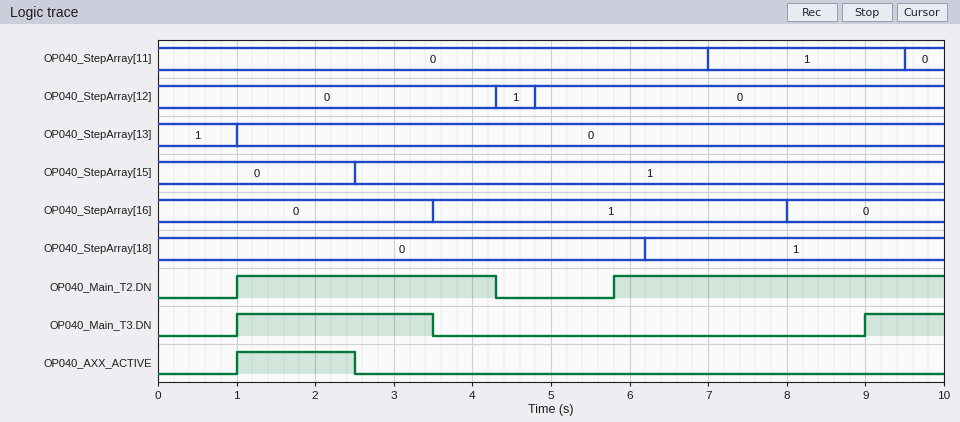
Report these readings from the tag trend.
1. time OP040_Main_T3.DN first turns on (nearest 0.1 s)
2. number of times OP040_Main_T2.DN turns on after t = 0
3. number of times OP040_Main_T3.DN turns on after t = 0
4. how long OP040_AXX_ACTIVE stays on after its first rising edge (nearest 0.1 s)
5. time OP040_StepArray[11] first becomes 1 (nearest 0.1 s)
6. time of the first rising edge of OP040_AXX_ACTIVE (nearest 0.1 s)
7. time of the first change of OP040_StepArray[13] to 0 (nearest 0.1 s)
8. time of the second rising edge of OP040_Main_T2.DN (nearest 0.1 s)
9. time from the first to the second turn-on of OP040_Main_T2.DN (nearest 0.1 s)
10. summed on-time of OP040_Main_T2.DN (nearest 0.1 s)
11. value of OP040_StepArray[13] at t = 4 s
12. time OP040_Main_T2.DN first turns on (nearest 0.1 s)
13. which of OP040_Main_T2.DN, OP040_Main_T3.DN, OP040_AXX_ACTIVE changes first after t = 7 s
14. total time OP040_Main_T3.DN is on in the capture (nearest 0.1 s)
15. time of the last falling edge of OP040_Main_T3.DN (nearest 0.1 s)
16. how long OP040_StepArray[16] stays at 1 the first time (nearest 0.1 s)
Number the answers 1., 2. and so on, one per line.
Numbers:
1. 1.0 s
2. 2
3. 2
4. 1.5 s
5. 7.0 s
6. 1.0 s
7. 1.0 s
8. 5.8 s
9. 4.8 s
10. 7.5 s
11. 0
12. 1.0 s
13. OP040_Main_T3.DN
14. 3.5 s
15. 3.5 s
16. 4.5 s
